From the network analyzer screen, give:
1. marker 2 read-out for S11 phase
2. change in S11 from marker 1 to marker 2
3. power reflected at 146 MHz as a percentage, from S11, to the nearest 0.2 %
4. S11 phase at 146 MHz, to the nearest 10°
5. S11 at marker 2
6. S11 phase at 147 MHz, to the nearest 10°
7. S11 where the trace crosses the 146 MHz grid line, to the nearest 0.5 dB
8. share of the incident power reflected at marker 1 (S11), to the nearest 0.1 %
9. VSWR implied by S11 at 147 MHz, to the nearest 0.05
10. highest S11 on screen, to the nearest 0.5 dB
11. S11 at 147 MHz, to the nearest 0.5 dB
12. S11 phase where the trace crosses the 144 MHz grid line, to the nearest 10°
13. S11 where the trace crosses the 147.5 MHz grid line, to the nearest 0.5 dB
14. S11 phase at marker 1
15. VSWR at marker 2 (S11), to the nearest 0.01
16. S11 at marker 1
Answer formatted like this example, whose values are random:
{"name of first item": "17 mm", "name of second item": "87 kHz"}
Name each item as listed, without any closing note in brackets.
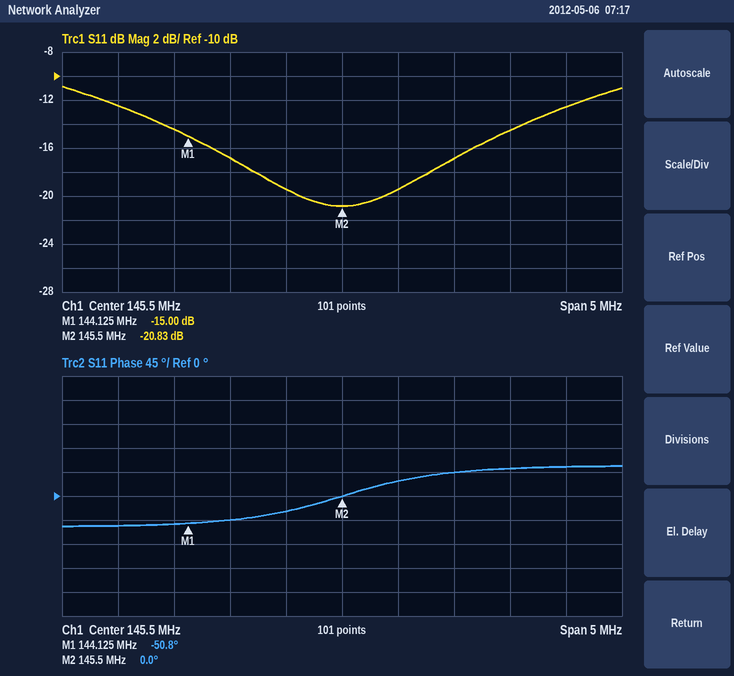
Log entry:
{"marker 2 read-out for S11 phase": "0.0°", "change in S11 from marker 1 to marker 2": "-5.83 dB", "power reflected at 146 MHz as a percentage, from S11, to the nearest 0.2 %": "1.2 %", "S11 phase at 146 MHz, to the nearest 10°": "30°", "S11 at marker 2": "-20.83 dB", "S11 phase at 147 MHz, to the nearest 10°": "50°", "S11 where the trace crosses the 146 MHz grid line, to the nearest 0.5 dB": "-19.5 dB", "share of the incident power reflected at marker 1 (S11), to the nearest 0.1 %": "3.2 %", "VSWR implied by S11 at 147 MHz, to the nearest 0.05": "1.45", "highest S11 on screen, to the nearest 0.5 dB": "-11.0 dB", "S11 at 147 MHz, to the nearest 0.5 dB": "-14.5 dB", "S11 phase where the trace crosses the 144 MHz grid line, to the nearest 10°": "-50°", "S11 where the trace crosses the 147.5 MHz grid line, to the nearest 0.5 dB": "-12.5 dB", "S11 phase at marker 1": "-50.8°", "VSWR at marker 2 (S11), to the nearest 0.01": "1.20", "S11 at marker 1": "-15.00 dB"}
